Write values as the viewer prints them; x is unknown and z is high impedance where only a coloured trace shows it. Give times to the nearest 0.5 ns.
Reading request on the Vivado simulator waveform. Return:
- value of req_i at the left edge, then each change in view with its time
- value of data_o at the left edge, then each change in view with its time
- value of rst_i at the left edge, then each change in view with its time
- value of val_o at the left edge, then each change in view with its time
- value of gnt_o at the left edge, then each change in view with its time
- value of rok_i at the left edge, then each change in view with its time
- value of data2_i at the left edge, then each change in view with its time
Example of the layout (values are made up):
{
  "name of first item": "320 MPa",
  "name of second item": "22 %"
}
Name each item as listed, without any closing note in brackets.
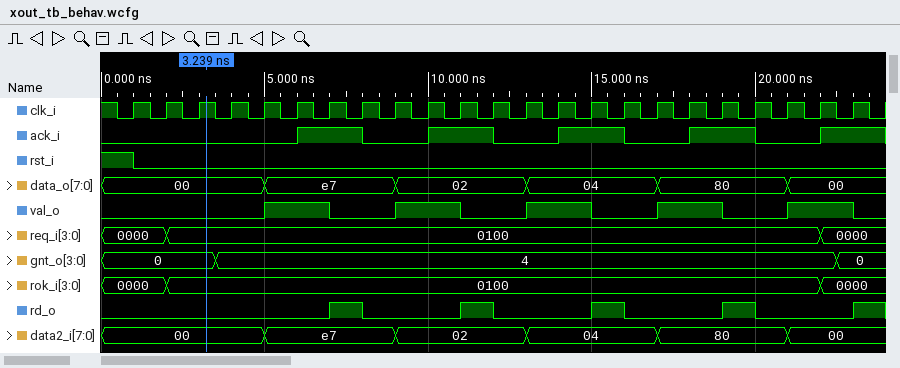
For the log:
{
  "value of req_i at the left edge, then each change in view with its time": "0000, 0100 at 2 ns, 0000 at 22 ns",
  "value of data_o at the left edge, then each change in view with its time": "00, e7 at 5 ns, 02 at 9 ns, 04 at 13 ns, 80 at 17 ns, 00 at 21 ns",
  "value of rst_i at the left edge, then each change in view with its time": "1, 0 at 1 ns",
  "value of val_o at the left edge, then each change in view with its time": "0, 1 at 5 ns, 0 at 7 ns, 1 at 9 ns, 0 at 11 ns, 1 at 13 ns, 0 at 15 ns, 1 at 17 ns, 0 at 19 ns, 1 at 21 ns, 0 at 23 ns",
  "value of gnt_o at the left edge, then each change in view with its time": "0, 4 at 3.5 ns, 0 at 22.5 ns",
  "value of rok_i at the left edge, then each change in view with its time": "0000, 0100 at 2 ns, 0000 at 22 ns",
  "value of data2_i at the left edge, then each change in view with its time": "00, e7 at 5 ns, 02 at 9 ns, 04 at 13 ns, 80 at 17 ns, 00 at 21 ns"
}
